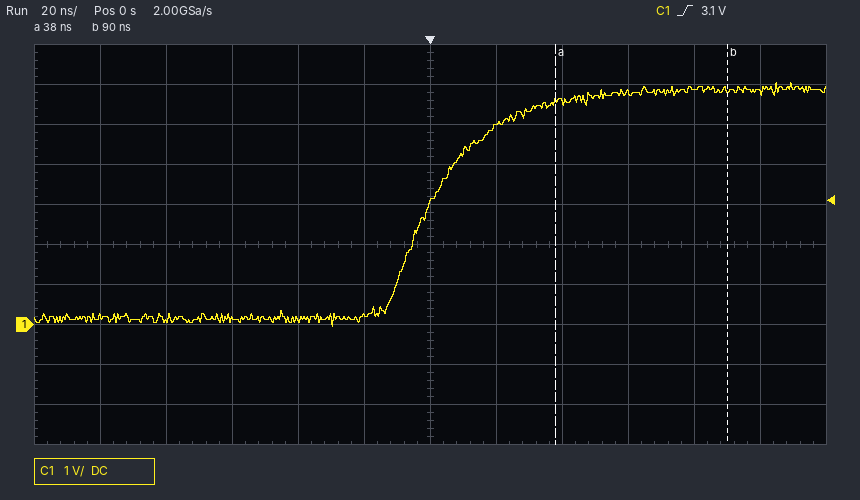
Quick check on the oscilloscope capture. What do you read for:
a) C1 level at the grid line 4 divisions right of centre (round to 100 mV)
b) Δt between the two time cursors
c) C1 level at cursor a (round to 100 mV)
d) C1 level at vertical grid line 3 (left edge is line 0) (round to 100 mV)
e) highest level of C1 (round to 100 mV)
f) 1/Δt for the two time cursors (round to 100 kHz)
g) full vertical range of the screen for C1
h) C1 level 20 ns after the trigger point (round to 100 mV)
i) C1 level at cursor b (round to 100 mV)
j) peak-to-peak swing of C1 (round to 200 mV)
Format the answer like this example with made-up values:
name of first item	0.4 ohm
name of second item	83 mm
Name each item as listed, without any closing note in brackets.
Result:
C1 level at the grid line 4 divisions right of centre	5.9 V
Δt between the two time cursors	52 ns
C1 level at cursor a	5.6 V
C1 level at vertical grid line 3 (left edge is line 0)	100 mV
highest level of C1	6.0 V
1/Δt for the two time cursors	19.2 MHz
full vertical range of the screen for C1	10 V
C1 level 20 ns after the trigger point	5.0 V
C1 level at cursor b	5.9 V
peak-to-peak swing of C1	6.0 V
